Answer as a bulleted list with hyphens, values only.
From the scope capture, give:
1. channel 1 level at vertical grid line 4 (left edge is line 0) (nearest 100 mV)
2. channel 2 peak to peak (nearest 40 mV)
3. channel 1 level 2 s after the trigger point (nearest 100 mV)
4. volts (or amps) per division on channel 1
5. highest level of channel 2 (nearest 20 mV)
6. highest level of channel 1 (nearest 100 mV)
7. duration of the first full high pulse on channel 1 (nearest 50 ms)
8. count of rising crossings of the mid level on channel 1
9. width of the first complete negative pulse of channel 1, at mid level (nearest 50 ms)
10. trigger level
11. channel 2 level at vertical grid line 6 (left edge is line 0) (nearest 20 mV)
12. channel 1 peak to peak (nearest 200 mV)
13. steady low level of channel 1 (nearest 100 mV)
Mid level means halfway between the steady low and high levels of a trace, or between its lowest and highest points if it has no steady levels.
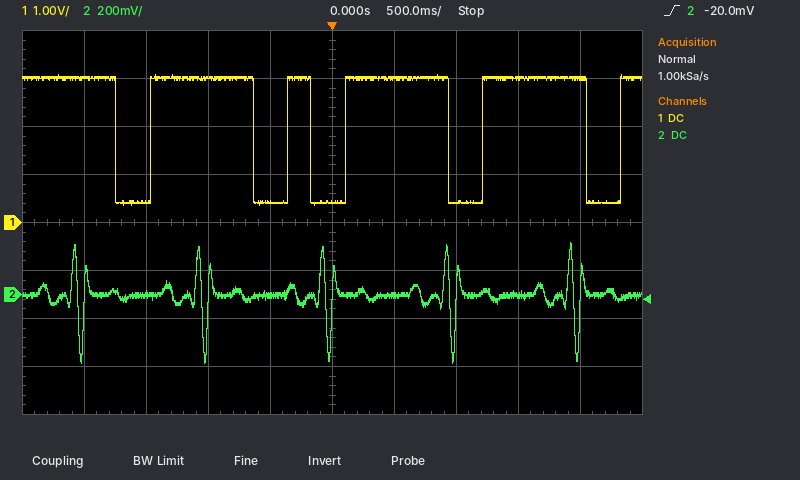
- 400 mV
- 520 mV
- 3.0 V
- 1 V
- 220 mV
- 3.1 V
- 850 ms
- 5
- 300 ms
- -20.0 mV
- 0 mV
- 2.8 V
- 400 mV
